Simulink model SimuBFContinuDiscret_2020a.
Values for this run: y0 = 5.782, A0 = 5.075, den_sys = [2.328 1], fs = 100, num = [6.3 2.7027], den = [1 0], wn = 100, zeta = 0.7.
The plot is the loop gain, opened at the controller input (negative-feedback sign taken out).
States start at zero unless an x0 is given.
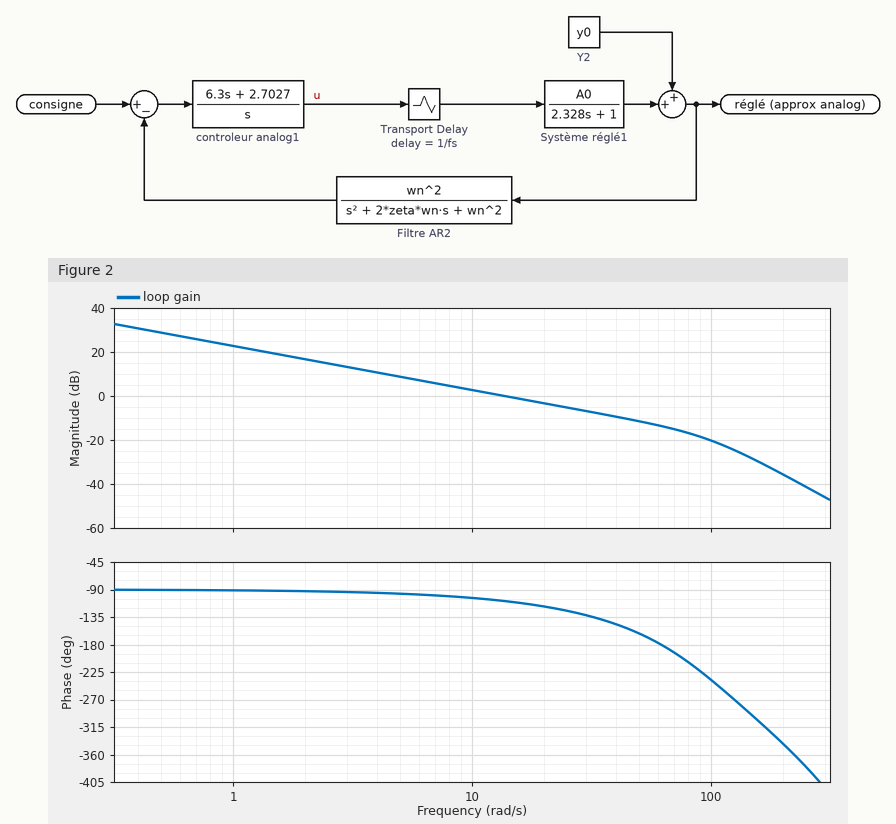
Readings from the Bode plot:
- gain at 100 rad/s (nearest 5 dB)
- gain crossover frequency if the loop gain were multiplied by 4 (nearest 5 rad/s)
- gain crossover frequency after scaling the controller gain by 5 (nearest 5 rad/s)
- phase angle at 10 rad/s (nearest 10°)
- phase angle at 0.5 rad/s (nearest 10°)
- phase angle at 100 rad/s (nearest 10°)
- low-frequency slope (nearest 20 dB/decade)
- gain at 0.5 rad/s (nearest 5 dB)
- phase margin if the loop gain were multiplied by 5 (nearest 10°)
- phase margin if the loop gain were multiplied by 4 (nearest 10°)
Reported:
-20 dB
55 rad/s
65 rad/s
-100°
-90°
-240°
-20 dB/decade
30 dB
0°
10°
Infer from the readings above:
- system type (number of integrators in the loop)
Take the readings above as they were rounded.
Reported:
1
